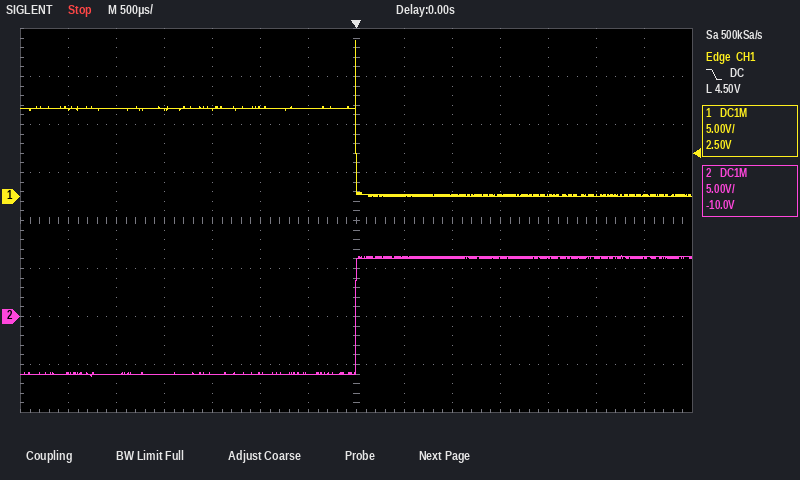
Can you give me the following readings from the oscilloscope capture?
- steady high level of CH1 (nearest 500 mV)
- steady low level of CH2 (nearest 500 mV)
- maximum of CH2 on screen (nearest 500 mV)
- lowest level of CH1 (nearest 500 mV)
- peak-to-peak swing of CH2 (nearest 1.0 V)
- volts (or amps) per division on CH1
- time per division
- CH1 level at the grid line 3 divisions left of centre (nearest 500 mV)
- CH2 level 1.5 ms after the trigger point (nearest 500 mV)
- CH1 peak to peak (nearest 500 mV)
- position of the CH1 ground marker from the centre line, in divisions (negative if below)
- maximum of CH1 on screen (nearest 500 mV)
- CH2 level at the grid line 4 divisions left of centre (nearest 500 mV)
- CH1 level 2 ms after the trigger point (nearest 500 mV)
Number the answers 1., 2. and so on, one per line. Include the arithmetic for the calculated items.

1. 9.0 V
2. -6.0 V
3. 6.5 V
4. 0.0 V
5. 13.0 V
6. 5 V
7. 500 µs
8. 9.0 V
9. 6.0 V
10. 16.0 V − (0.0 V) = 16.0 V
11. +0.5 div
12. 16.0 V
13. -6.0 V
14. 0.0 V
